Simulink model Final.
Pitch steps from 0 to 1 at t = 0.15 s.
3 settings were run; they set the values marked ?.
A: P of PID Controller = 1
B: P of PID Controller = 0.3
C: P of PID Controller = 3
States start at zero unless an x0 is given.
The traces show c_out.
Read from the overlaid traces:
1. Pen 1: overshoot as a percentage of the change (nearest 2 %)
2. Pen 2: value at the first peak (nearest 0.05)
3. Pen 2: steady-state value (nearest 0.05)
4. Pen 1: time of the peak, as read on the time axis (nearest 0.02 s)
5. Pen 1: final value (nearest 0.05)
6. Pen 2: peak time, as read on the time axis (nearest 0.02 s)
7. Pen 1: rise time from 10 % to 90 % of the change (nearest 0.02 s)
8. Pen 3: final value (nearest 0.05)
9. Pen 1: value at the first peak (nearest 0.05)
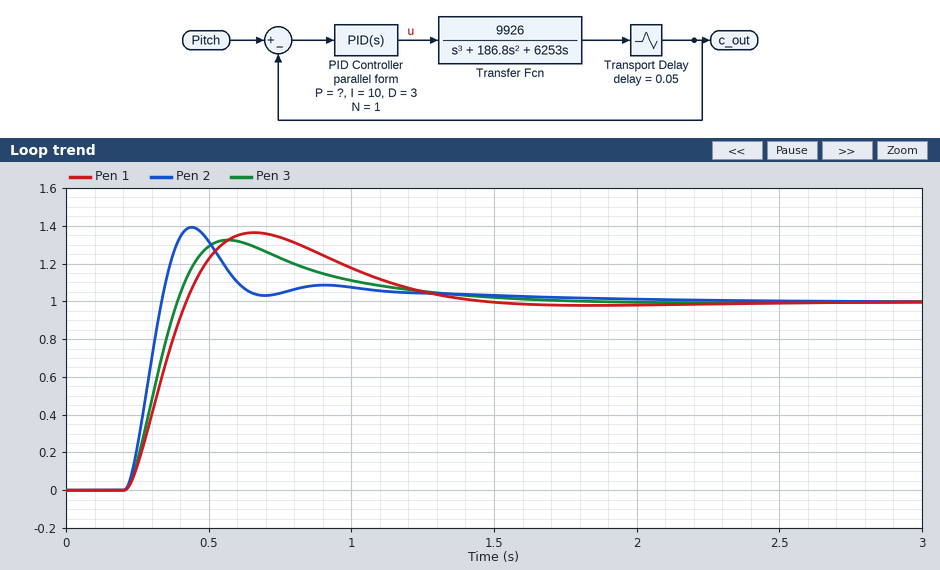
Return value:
36 %
1.40
1.00
0.66 s
1.00
0.44 s
0.16 s
1.00
1.35
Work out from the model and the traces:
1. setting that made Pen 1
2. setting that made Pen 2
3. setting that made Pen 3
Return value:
B
C
A
